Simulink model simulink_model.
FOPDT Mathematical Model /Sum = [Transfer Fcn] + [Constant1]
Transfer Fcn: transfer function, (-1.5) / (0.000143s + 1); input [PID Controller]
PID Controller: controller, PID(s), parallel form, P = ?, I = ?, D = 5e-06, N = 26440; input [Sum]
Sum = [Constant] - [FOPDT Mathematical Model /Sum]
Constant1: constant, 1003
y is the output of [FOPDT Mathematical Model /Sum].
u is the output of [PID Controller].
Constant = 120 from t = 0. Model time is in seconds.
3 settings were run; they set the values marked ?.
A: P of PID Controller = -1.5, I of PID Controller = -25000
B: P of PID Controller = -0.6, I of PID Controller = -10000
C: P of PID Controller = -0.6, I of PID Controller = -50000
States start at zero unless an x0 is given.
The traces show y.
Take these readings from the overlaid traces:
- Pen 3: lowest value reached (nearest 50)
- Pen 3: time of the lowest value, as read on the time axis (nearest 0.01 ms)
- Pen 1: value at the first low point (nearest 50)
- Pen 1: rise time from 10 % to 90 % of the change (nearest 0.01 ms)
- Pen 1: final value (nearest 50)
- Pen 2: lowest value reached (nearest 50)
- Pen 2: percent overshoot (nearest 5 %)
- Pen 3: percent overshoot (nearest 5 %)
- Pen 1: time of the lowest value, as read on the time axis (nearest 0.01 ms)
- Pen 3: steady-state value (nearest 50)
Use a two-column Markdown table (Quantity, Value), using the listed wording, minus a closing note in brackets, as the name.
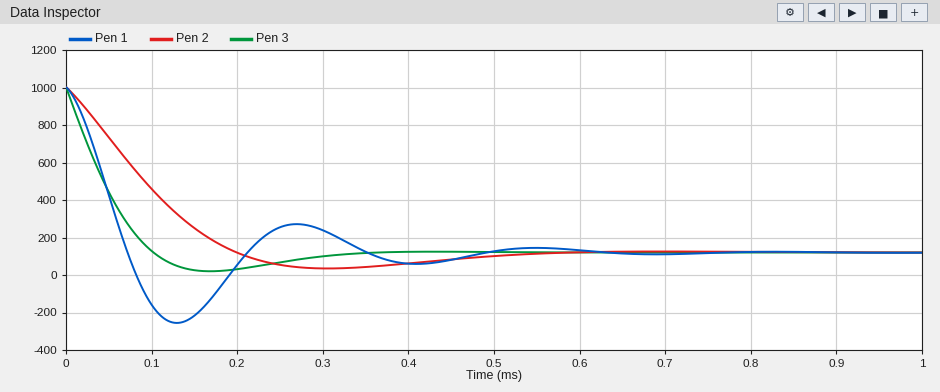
| Quantity | Value |
|---|---|
| Pen 3: lowest value reached | 0 |
| Pen 3: time of the lowest value, as read on the time axis | 0.17 ms |
| Pen 1: value at the first low point | -250 |
| Pen 1: rise time from 10 % to 90 % of the change | 0.05 ms |
| Pen 1: final value | 100 |
| Pen 2: lowest value reached | 50 |
| Pen 2: percent overshoot | 10 % |
| Pen 3: percent overshoot | 10 % |
| Pen 1: time of the lowest value, as read on the time axis | 0.13 ms |
| Pen 3: steady-state value | 100 |
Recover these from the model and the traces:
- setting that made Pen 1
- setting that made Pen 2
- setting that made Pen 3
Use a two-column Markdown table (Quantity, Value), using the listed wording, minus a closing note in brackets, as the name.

| Quantity | Value |
|---|---|
| setting that made Pen 1 | C |
| setting that made Pen 2 | B |
| setting that made Pen 3 | A |
